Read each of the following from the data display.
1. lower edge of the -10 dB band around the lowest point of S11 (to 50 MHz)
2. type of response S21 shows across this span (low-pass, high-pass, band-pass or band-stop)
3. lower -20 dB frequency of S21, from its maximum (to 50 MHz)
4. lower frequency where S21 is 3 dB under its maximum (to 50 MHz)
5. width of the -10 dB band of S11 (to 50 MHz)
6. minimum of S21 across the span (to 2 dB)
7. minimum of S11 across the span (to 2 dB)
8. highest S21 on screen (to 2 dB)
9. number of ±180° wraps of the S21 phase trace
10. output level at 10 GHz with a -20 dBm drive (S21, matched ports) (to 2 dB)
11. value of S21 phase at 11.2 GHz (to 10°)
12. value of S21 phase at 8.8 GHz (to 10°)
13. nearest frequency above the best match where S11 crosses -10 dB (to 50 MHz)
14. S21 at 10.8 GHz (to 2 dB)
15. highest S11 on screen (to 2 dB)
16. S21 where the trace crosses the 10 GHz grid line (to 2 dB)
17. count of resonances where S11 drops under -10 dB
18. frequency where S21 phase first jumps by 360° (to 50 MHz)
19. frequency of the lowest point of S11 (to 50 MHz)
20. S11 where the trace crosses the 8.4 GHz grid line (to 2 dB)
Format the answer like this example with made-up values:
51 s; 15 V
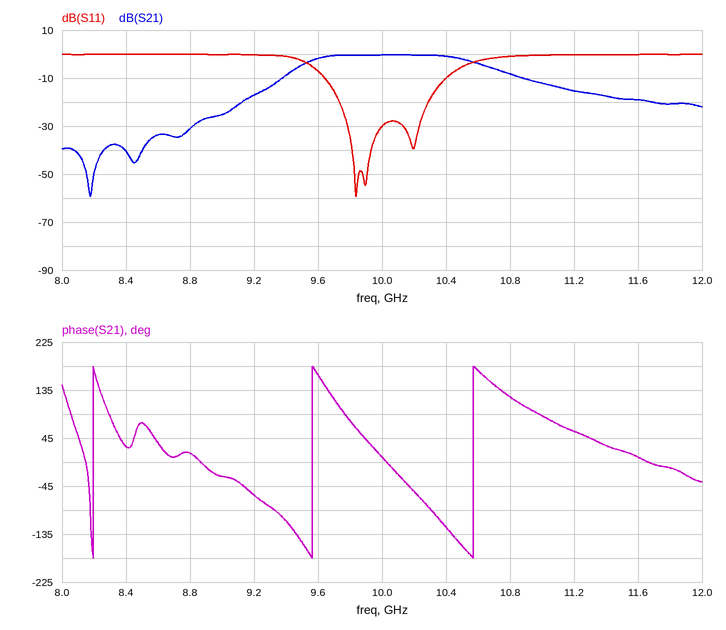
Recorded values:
9.65 GHz; band-pass; 9.10 GHz; 9.55 GHz; 750 MHz; -60 dB; -60 dB; 0 dB; 3; -20 dBm; 60°; 20°; 10.40 GHz; -8 dB; 0 dB; 0 dB; 3; 8.20 GHz; 9.85 GHz; 0 dB
